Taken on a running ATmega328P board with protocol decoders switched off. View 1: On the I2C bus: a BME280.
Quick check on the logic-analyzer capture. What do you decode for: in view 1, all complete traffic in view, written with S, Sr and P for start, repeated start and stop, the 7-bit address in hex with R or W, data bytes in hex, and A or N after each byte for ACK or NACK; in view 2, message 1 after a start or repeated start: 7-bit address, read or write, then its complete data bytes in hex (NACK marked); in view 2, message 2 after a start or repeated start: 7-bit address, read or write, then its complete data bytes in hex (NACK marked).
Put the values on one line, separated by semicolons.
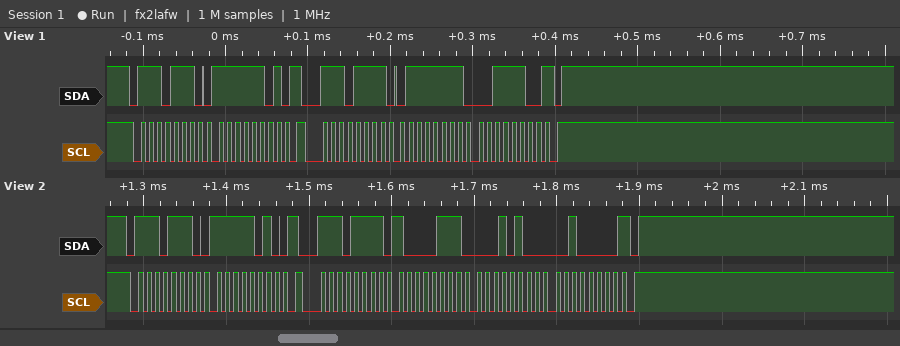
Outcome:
S 77W A FD A Sr 77R A 7F A 3C N P; 0x77 write: FA; 0x77 read: 87 14 20 NACK
